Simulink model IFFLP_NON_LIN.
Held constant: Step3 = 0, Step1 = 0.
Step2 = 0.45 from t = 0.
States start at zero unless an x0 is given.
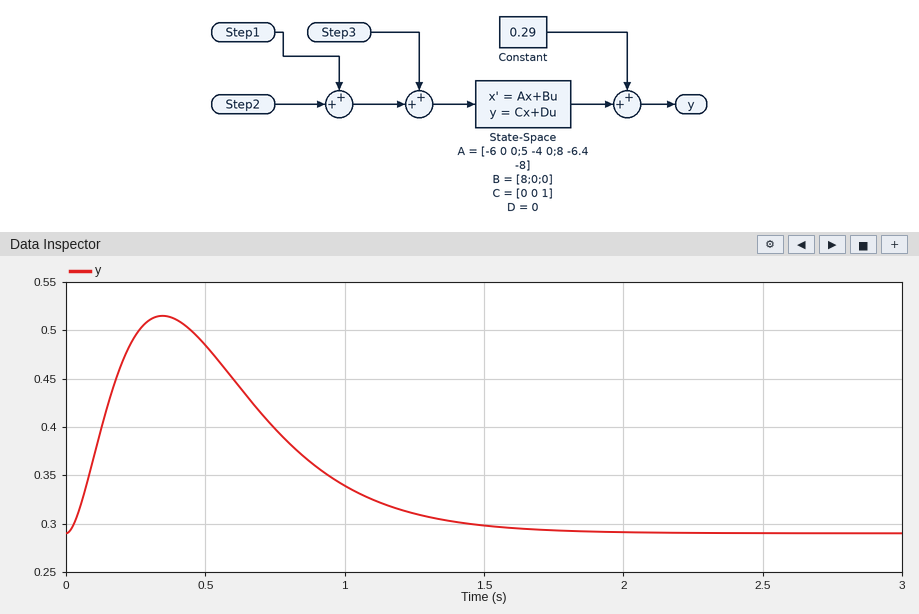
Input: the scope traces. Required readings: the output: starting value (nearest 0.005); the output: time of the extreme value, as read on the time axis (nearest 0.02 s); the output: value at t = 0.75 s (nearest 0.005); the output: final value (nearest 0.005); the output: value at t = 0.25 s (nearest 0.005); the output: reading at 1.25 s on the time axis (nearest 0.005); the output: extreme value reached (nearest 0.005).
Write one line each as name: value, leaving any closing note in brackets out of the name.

the output: starting value: 0.290
the output: time of the extreme value, as read on the time axis: 0.34 s
the output: value at t = 0.75 s: 0.400
the output: final value: 0.290
the output: value at t = 0.25 s: 0.495
the output: reading at 1.25 s on the time axis: 0.310
the output: extreme value reached: 0.515
